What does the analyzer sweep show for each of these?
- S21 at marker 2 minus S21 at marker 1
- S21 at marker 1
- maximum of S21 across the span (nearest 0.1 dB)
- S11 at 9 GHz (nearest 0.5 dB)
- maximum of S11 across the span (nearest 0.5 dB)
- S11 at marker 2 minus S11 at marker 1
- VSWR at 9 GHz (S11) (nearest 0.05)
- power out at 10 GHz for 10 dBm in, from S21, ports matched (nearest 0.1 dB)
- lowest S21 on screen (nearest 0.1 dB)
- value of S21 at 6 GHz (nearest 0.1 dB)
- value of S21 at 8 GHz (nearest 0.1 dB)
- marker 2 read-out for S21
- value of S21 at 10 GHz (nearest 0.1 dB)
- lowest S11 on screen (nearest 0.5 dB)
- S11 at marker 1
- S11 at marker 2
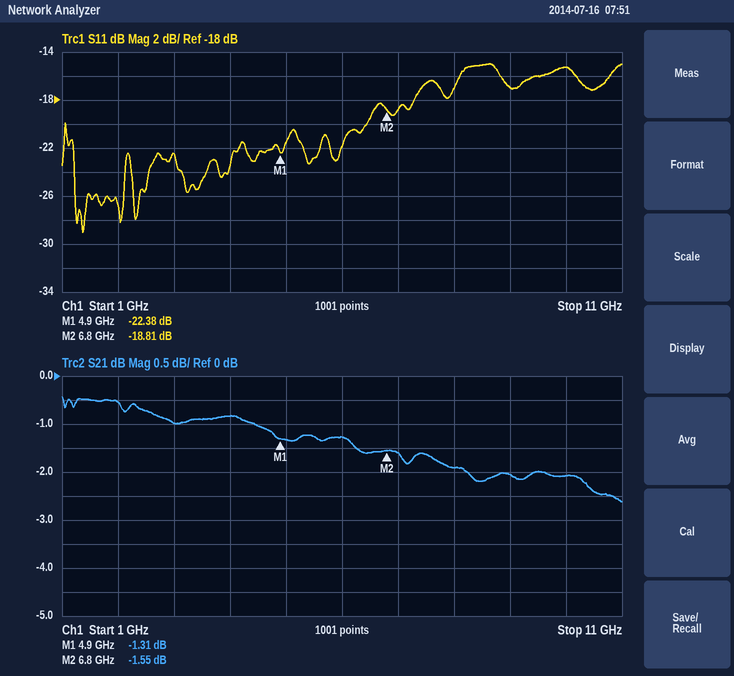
-0.24 dB
-1.31 dB
-0.4 dB
-17.0 dB
-15.0 dB
3.57 dB
1.35
7.9 dBm
-2.6 dB
-1.3 dB
-1.9 dB
-1.55 dB
-2.1 dB
-29.0 dB
-22.38 dB
-18.81 dB
